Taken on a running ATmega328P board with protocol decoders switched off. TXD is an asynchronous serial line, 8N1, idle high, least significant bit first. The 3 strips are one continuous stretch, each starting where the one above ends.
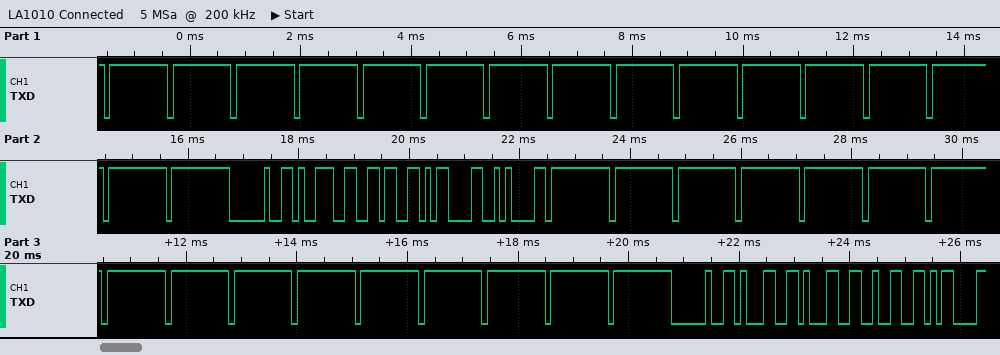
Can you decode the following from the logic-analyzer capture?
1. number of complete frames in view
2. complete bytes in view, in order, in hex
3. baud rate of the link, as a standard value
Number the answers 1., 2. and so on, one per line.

1. 42
2. FF FF FF FF FF FF FF FF FF FF FF FF FF FF FF FF 20 39 36 0D 0A FF FF FF FF FF FF FF FF FF FF FF FF FF FF FF FF 20 31 31 32 0D
3. 9600 baud
